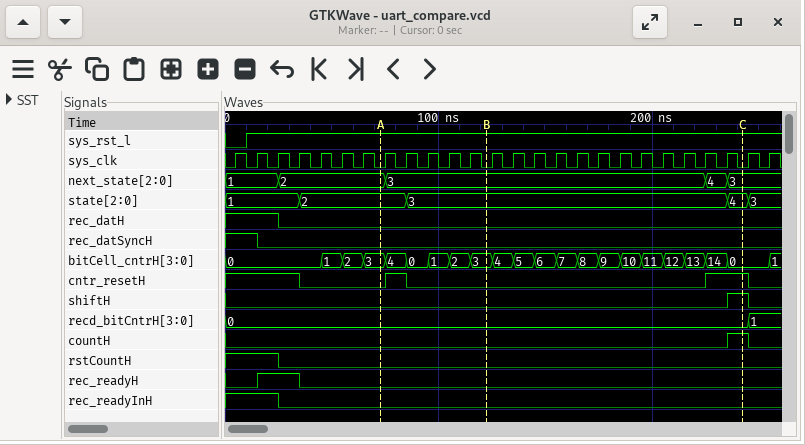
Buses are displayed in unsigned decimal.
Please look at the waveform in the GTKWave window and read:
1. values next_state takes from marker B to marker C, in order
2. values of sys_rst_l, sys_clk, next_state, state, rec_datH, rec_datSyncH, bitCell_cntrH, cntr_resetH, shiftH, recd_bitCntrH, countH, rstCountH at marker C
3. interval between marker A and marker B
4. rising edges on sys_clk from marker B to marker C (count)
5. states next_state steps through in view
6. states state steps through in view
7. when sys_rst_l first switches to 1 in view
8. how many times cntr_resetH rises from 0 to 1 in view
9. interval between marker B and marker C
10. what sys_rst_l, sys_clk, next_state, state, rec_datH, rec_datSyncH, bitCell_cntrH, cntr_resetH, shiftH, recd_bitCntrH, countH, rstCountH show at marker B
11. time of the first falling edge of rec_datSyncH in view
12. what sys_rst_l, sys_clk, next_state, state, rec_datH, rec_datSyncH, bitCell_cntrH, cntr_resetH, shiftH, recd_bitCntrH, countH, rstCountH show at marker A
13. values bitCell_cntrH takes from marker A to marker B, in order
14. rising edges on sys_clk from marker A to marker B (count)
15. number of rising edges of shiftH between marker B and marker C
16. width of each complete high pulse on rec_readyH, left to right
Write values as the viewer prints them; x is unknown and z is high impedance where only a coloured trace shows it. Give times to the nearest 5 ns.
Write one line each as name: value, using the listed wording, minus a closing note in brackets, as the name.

values next_state takes from marker B to marker C, in order: 3, 4, 3
values of sys_rst_l, sys_clk, next_state, state, rec_datH, rec_datSyncH, bitCell_cntrH, cntr_resetH, shiftH, recd_bitCntrH, countH, rstCountH at marker C: sys_rst_l=1, sys_clk=0, next_state=3, state=4, rec_datH=0, rec_datSyncH=0, bitCell_cntrH=0, cntr_resetH=1, shiftH=1, recd_bitCntrH=0, countH=1, rstCountH=0
interval between marker A and marker B: 50 ns
rising edges on sys_clk from marker B to marker C: 12
states next_state steps through in view: 1, 2, 3, 4, 3
states state steps through in view: 1, 2, 3, 4, 3
when sys_rst_l first switches to 1 in view: 10 ns
how many times cntr_resetH rises from 0 to 1 in view: 2
interval between marker B and marker C: 120 ns
what sys_rst_l, sys_clk, next_state, state, rec_datH, rec_datSyncH, bitCell_cntrH, cntr_resetH, shiftH, recd_bitCntrH, countH, rstCountH show at marker B: sys_rst_l=1, sys_clk=0, next_state=3, state=3, rec_datH=0, rec_datSyncH=0, bitCell_cntrH=3, cntr_resetH=0, shiftH=0, recd_bitCntrH=0, countH=0, rstCountH=0
time of the first falling edge of rec_datSyncH in view: 15 ns
what sys_rst_l, sys_clk, next_state, state, rec_datH, rec_datSyncH, bitCell_cntrH, cntr_resetH, shiftH, recd_bitCntrH, countH, rstCountH show at marker A: sys_rst_l=1, sys_clk=0, next_state=2, state=2, rec_datH=0, rec_datSyncH=0, bitCell_cntrH=3, cntr_resetH=0, shiftH=0, recd_bitCntrH=0, countH=0, rstCountH=0
values bitCell_cntrH takes from marker A to marker B, in order: 3, 4, 0, 1, 2, 3
rising edges on sys_clk from marker A to marker B: 5
number of rising edges of shiftH between marker B and marker C: 1
width of each complete high pulse on rec_readyH, left to right: 20 ns
